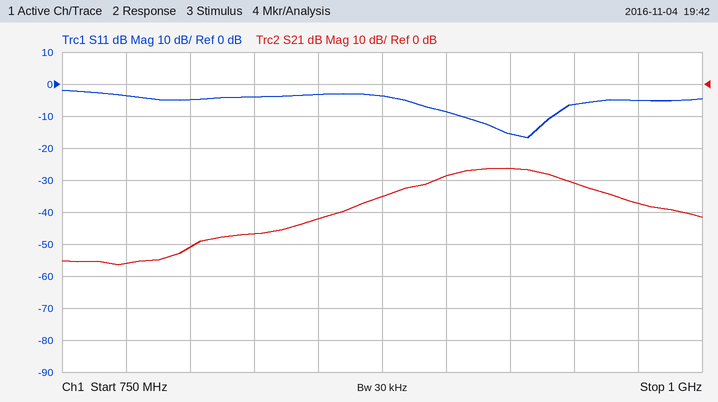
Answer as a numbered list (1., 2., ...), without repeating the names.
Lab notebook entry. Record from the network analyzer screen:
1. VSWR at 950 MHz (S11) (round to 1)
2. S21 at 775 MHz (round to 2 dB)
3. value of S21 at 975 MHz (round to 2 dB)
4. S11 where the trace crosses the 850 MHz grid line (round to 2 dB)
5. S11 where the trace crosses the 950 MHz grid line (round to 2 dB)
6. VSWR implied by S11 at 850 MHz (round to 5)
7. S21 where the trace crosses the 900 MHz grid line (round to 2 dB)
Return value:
1. 3
2. -56 dB
3. -38 dB
4. -4 dB
5. -6 dB
6. 5
7. -28 dB
